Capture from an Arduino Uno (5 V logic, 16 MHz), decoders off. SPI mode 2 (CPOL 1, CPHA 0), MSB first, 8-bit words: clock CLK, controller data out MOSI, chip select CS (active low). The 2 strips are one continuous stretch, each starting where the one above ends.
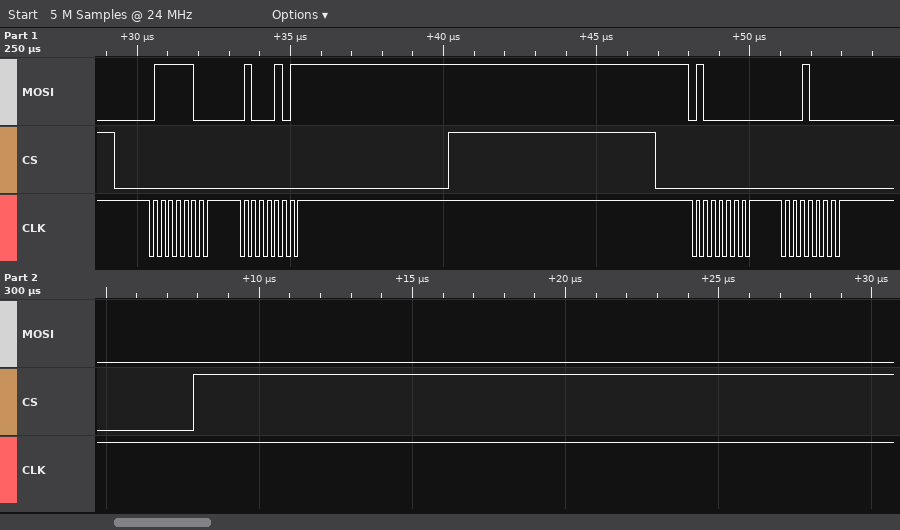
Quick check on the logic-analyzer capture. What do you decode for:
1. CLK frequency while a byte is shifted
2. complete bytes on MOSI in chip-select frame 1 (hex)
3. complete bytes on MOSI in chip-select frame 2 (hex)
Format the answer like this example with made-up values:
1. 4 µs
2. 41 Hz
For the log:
1. 4 MHz
2. 0x7C 0x45
3. 0x40 0x10
